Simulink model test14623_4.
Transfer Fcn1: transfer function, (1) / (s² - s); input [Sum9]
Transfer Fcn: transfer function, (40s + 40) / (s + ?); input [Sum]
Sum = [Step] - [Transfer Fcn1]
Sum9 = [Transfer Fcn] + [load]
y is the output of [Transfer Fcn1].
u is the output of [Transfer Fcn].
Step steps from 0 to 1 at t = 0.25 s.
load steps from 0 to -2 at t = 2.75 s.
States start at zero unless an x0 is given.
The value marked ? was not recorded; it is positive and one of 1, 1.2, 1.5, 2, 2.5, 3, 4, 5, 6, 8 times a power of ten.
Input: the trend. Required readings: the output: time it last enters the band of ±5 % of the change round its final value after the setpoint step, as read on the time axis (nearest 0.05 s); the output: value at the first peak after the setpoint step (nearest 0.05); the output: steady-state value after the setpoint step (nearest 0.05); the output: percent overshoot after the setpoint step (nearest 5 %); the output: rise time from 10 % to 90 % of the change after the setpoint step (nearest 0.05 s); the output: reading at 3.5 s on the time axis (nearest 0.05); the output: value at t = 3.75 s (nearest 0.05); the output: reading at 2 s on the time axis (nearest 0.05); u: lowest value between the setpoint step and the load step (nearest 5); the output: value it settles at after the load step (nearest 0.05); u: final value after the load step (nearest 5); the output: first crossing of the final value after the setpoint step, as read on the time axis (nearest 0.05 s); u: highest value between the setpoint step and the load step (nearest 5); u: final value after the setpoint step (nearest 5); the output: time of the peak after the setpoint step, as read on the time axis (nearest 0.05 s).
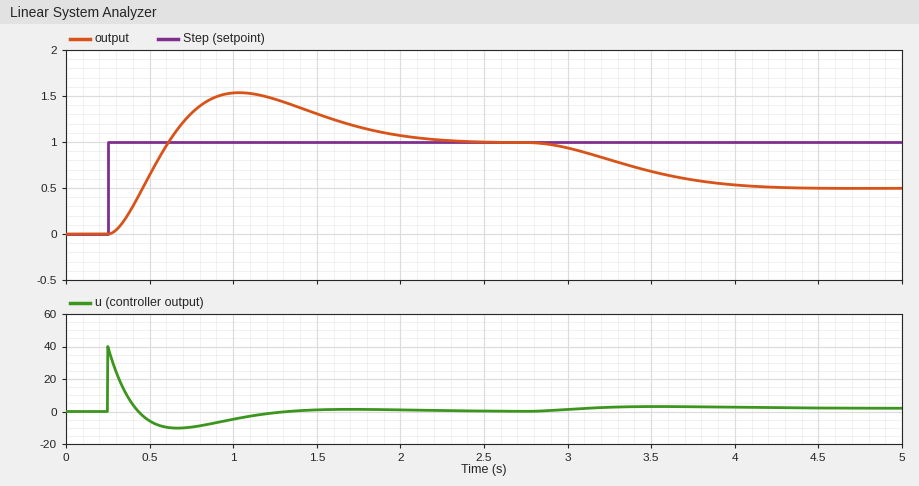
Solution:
2.10 s
1.55
1.00
55 %
0.25 s
0.70
0.60
1.05
-10
0.50
0
0.60 s
40
0
1.05 s
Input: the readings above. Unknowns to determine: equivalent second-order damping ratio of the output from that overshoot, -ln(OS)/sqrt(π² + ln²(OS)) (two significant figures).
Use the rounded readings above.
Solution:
0.19
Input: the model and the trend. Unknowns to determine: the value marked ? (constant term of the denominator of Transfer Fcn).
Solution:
10
